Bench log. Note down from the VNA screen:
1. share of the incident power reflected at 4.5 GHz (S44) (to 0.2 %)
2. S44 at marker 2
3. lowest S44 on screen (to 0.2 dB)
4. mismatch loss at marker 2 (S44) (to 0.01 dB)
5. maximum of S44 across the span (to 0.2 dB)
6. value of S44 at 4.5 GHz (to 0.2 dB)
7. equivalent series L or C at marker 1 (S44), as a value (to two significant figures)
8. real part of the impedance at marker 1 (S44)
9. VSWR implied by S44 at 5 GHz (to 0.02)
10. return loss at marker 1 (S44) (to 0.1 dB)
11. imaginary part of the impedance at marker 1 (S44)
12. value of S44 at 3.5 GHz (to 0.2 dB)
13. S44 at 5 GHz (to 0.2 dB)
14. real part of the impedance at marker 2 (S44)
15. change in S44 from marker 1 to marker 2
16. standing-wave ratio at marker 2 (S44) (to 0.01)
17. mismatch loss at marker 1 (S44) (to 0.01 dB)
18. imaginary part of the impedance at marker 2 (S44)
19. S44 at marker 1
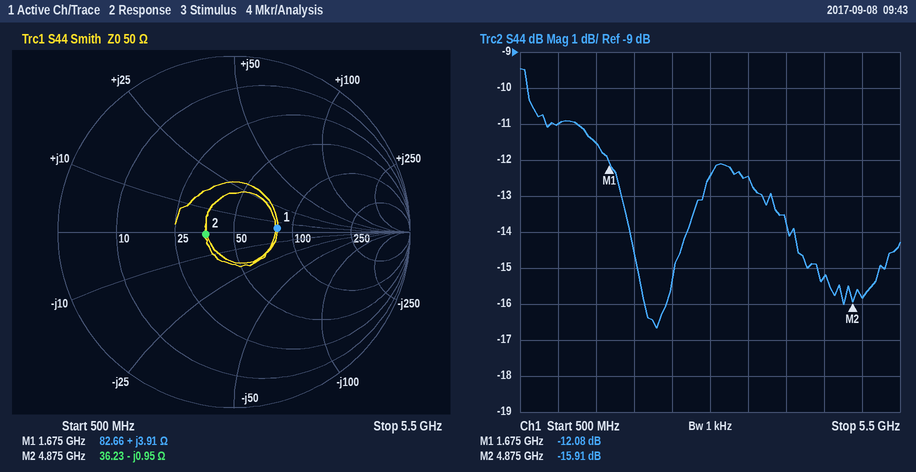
3.0 %
-15.91 dB
-16.6 dB
0.11 dB
-9.4 dB
-15.2 dB
370 pH
82.66 Ω
1.38
12.1 dB
+3.91 Ω
-12.4 dB
-15.8 dB
36.23 Ω
-3.83 dB
1.38
0.28 dB
-0.95 Ω
-12.08 dB
